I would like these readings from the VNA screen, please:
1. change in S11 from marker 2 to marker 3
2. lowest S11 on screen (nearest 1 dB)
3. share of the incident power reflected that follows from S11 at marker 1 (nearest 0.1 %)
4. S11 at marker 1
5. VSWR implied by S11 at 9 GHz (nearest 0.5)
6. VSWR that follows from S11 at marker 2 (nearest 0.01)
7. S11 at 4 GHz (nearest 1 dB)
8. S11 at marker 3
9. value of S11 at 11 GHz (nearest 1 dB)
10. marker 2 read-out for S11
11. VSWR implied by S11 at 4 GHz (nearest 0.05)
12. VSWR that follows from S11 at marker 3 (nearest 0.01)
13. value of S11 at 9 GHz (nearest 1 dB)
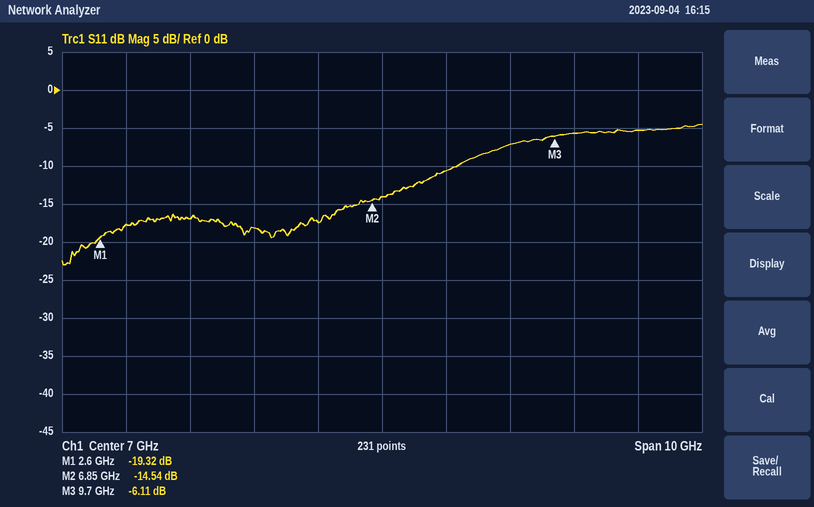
8.43 dB
-23 dB
1.2 %
-19.32 dB
2.5
1.46
-17 dB
-6.11 dB
-5 dB
-14.54 dB
1.35
2.96
-7 dB
